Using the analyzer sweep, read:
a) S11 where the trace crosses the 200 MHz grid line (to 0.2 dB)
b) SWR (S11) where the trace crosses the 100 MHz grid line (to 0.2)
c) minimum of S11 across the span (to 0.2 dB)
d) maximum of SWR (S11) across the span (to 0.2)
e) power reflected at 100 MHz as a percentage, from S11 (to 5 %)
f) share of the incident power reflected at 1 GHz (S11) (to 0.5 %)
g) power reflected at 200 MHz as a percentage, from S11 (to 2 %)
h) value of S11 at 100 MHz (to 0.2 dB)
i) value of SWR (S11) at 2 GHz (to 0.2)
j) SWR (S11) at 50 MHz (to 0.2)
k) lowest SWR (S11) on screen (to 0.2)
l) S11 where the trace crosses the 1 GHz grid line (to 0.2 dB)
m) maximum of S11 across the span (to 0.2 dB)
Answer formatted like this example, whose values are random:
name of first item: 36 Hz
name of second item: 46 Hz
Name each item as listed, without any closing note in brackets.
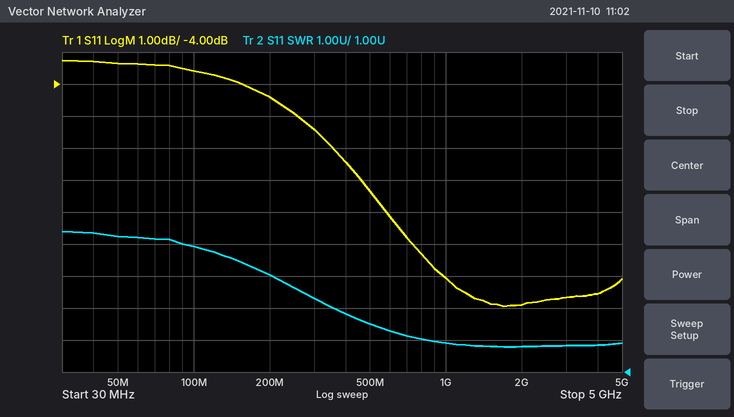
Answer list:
S11 where the trace crosses the 200 MHz grid line: -4.4 dB
SWR (S11) where the trace crosses the 100 MHz grid line: 5.0
minimum of S11 across the span: -11.0 dB
maximum of SWR (S11) across the span: 5.4
power reflected at 100 MHz as a percentage, from S11: 45 %
share of the incident power reflected at 1 GHz (S11): 10.0 %
power reflected at 200 MHz as a percentage, from S11: 36 %
value of S11 at 100 MHz: -3.6 dB
value of SWR (S11) at 2 GHz: 1.8
SWR (S11) at 50 MHz: 5.2
lowest SWR (S11) on screen: 1.8
S11 where the trace crosses the 1 GHz grid line: -10.0 dB
maximum of S11 across the span: -3.2 dB
